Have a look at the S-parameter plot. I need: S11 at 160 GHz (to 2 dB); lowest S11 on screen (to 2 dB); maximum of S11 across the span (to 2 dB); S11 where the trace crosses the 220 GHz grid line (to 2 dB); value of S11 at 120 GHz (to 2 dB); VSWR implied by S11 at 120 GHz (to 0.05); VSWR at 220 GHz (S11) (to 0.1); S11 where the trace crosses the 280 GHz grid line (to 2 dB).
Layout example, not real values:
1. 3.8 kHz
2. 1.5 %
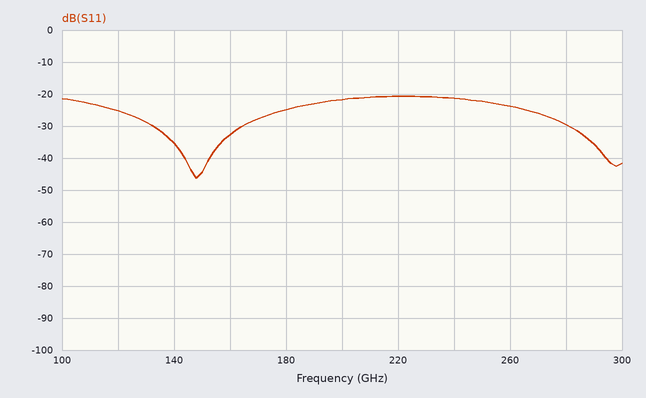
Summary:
1. -32 dB
2. -46 dB
3. -20 dB
4. -20 dB
5. -26 dB
6. 1.10
7. 1.2
8. -30 dB
